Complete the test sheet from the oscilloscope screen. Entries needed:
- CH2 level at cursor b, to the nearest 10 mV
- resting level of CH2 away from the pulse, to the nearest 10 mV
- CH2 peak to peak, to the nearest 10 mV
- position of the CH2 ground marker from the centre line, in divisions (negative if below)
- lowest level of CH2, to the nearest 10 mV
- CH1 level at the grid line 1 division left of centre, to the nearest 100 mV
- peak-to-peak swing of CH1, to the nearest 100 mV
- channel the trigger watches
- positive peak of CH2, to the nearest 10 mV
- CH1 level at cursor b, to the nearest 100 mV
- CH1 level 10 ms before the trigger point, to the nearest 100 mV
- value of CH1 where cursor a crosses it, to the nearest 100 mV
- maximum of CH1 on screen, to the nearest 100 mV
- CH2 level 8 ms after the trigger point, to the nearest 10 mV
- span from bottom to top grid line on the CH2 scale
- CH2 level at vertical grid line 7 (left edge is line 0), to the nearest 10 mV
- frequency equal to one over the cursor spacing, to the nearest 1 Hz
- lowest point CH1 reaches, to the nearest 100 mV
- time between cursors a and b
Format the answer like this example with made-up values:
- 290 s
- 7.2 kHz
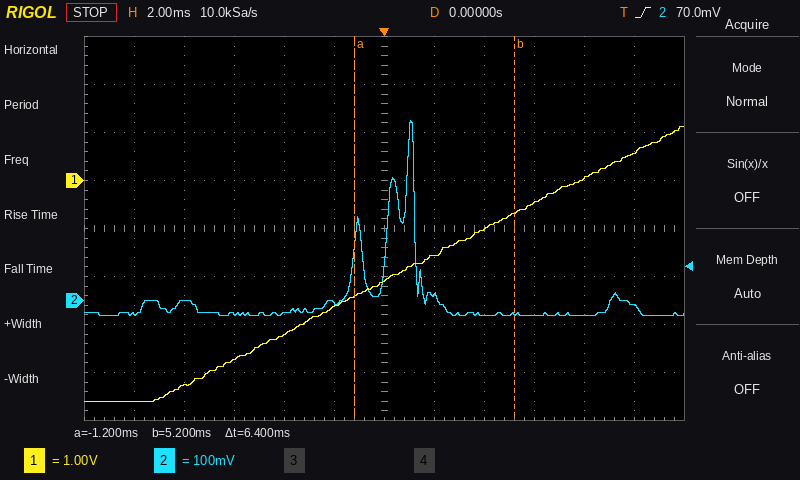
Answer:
- -30 mV
- -30 mV
- 410 mV
- -1.5 div
- -30 mV
- -2.6 V
- 5.7 V
- CH2
- 380 mV
- -700 mV
- -4.6 V
- -2.4 V
- 1.1 V
- -30 mV
- 800 mV
- 10 mV
- 156 Hz
- -4.6 V
- 6.4 ms
